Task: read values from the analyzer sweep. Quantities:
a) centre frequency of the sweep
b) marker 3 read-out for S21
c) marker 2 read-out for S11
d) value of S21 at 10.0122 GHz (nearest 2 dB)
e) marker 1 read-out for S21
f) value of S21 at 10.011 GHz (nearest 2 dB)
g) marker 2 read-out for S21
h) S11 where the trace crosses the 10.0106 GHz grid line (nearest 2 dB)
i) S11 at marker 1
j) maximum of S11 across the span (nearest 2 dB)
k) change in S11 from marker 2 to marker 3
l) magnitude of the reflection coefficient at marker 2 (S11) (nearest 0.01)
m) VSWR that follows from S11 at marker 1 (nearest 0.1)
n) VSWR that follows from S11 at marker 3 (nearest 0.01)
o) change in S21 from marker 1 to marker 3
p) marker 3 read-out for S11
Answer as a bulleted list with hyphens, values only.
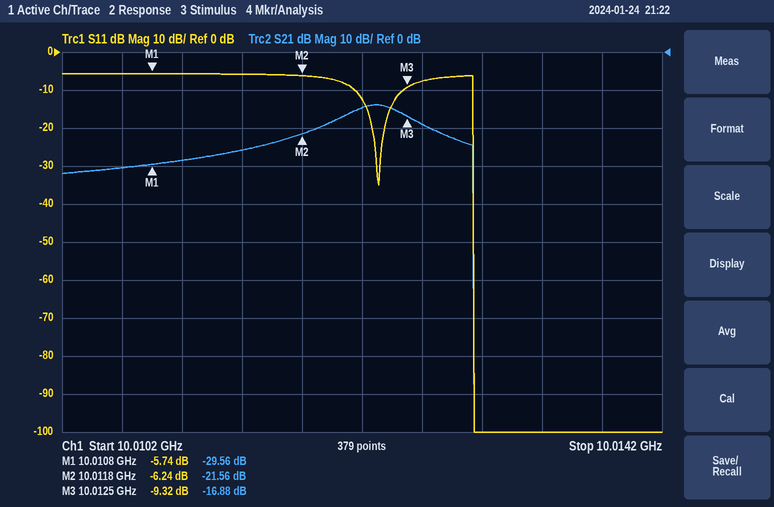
- 10.0122 GHz
- -16.88 dB
- -6.24 dB
- -14 dB
- -29.56 dB
- -28 dB
- -21.56 dB
- -6 dB
- -5.74 dB
- -6 dB
- -3.08 dB
- 0.49
- 3.1
- 2.04
- 12.68 dB
- -9.32 dB
